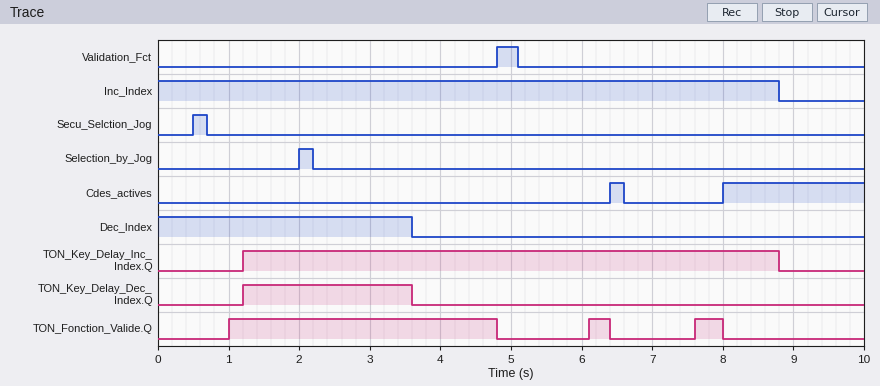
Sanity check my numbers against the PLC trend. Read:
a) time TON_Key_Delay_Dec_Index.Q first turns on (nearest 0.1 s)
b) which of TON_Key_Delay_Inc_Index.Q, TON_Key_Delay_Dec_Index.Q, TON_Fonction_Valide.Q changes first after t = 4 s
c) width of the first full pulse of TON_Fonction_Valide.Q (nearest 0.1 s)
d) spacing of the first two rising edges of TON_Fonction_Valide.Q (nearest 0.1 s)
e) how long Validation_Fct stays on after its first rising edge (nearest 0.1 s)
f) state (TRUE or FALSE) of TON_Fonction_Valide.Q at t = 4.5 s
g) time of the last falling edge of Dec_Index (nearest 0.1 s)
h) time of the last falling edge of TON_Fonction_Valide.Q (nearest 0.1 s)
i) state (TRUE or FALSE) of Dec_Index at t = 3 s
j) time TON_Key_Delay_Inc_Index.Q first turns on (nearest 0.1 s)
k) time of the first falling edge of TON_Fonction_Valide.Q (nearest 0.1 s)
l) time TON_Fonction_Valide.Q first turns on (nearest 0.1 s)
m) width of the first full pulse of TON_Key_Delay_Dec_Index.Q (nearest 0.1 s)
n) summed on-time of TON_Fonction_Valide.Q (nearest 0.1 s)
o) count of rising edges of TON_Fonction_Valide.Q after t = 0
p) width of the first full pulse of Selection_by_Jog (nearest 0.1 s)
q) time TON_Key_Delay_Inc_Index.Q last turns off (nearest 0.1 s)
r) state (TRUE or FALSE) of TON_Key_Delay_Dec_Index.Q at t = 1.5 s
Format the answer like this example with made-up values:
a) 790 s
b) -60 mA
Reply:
a) 1.2 s
b) TON_Fonction_Valide.Q
c) 3.8 s
d) 5.1 s
e) 0.3 s
f) TRUE
g) 3.6 s
h) 8.0 s
i) TRUE
j) 1.2 s
k) 4.8 s
l) 1.0 s
m) 2.4 s
n) 4.5 s
o) 3
p) 0.2 s
q) 8.8 s
r) TRUE
